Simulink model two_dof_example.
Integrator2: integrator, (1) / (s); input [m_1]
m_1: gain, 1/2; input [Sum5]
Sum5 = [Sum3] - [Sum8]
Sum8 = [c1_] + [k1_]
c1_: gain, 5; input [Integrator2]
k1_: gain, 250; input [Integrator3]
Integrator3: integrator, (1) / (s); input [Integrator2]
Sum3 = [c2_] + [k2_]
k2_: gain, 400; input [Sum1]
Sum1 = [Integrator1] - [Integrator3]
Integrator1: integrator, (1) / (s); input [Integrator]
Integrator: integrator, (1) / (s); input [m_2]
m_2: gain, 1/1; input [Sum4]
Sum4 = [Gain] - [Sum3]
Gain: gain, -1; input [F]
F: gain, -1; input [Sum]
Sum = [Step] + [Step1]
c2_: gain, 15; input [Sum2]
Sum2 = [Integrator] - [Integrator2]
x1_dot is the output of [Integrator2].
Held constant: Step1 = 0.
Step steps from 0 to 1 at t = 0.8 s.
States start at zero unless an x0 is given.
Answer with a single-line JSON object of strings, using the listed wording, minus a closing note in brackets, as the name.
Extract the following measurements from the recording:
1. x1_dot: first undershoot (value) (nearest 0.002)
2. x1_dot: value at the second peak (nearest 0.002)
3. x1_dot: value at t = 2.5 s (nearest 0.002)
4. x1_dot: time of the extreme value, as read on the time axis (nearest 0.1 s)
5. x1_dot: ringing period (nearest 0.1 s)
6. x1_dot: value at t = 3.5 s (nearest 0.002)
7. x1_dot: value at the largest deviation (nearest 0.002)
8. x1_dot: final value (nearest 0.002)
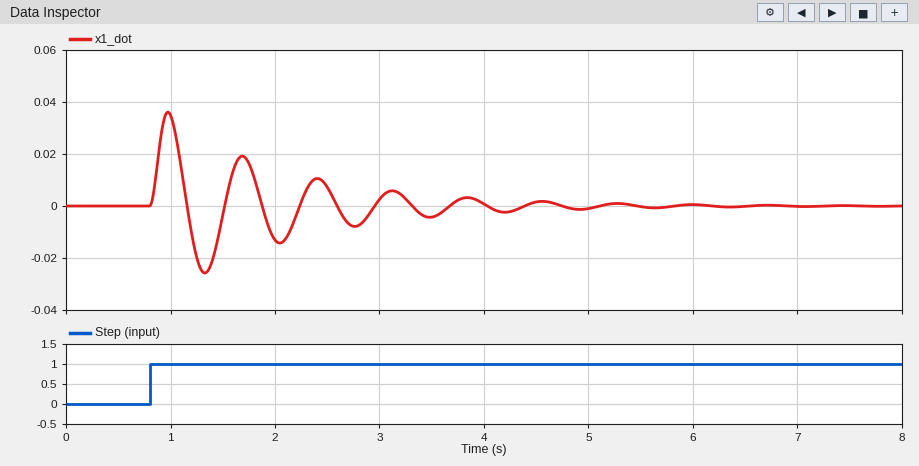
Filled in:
{"x1_dot: first undershoot (value)": "-0.026", "x1_dot: value at the second peak": "0.020", "x1_dot: value at t = 2.5 s": "0.008", "x1_dot: time of the extreme value, as read on the time axis": "1.0 s", "x1_dot: ringing period": "0.7 s", "x1_dot: value at t = 3.5 s": "-0.004", "x1_dot: value at the largest deviation": "0.036", "x1_dot: final value": "0.000"}
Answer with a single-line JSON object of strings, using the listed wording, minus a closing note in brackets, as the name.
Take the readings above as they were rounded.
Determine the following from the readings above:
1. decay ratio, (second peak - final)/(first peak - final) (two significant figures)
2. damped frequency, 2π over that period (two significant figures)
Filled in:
{"decay ratio, (second peak - final)/(first peak - final)": "0.56", "damped frequency, 2π over that period": "9.0 rad/s"}
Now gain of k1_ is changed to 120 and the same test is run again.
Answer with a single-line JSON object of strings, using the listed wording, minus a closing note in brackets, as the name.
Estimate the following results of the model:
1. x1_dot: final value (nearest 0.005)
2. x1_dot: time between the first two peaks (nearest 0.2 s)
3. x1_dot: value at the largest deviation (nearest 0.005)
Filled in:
{"x1_dot: final value": "0.000", "x1_dot: time between the first two peaks": "1.0 s", "x1_dot: value at the largest deviation": "0.045"}
